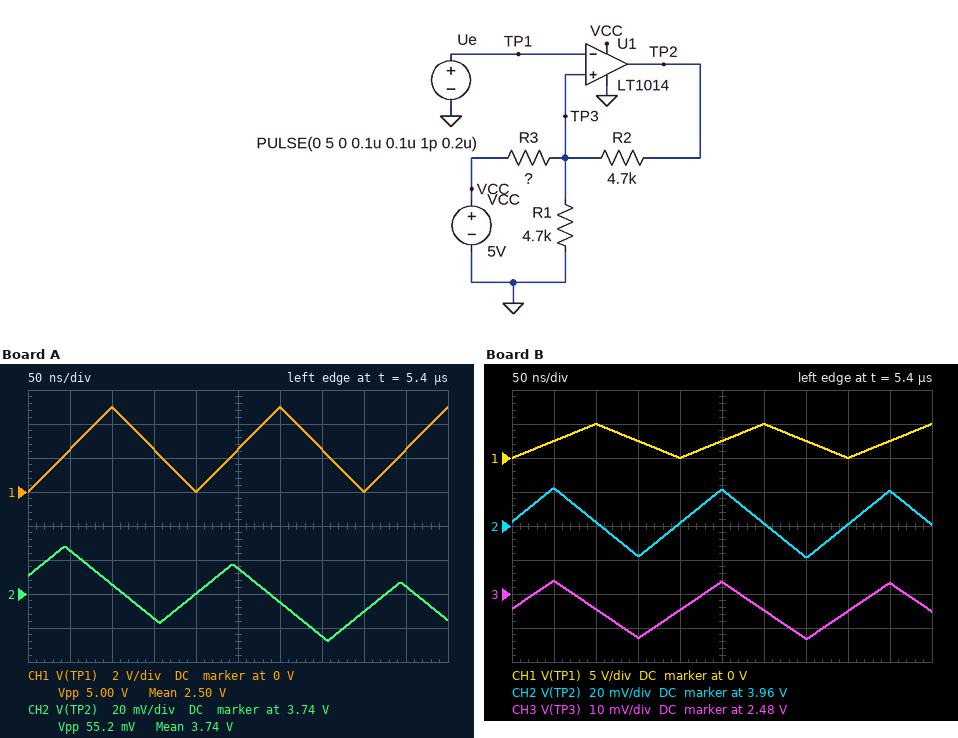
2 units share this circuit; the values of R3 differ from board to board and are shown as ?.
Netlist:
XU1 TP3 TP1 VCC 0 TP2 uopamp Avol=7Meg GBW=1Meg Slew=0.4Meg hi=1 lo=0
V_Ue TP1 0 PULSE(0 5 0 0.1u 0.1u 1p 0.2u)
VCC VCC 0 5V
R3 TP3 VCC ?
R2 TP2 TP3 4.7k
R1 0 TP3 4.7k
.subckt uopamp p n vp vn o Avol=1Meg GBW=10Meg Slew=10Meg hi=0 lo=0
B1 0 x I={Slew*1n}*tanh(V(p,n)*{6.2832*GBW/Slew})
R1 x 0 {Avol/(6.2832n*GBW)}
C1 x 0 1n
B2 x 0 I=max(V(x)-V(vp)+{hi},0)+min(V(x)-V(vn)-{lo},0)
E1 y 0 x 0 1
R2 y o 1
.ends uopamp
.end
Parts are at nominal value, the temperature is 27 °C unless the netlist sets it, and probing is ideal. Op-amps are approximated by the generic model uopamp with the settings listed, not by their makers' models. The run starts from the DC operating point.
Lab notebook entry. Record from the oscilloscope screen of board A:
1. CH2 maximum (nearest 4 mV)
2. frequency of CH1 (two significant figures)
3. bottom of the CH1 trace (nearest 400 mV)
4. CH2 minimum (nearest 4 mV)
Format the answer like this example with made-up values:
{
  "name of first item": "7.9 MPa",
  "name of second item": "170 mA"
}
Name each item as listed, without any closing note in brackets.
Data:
{
  "CH2 maximum": "3.768 V",
  "frequency of CH1": "5.0 MHz",
  "bottom of the CH1 trace": "0 V",
  "CH2 minimum": "3.712 V"
}
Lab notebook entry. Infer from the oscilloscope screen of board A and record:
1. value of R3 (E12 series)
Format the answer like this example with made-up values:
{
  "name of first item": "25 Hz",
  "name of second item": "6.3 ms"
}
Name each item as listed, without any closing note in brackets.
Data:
{
  "value of R3": "22 kΩ"
}
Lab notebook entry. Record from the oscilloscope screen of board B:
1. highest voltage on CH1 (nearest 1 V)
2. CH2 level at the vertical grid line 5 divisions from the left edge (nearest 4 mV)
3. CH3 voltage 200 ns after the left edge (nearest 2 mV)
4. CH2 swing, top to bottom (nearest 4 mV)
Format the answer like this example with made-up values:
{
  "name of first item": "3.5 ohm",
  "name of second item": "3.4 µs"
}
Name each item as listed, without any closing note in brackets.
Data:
{
  "highest voltage on CH1": "5 V",
  "CH2 level at the vertical grid line 5 divisions from the left edge": "3.980 V",
  "CH3 voltage 200 ns after the left edge": "2.476 V",
  "CH2 swing, top to bottom": "40 mV"
}
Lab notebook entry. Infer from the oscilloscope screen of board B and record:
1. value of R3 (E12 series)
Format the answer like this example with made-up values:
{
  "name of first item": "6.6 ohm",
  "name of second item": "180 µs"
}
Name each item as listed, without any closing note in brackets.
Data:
{
  "value of R3": "12 kΩ"
}
